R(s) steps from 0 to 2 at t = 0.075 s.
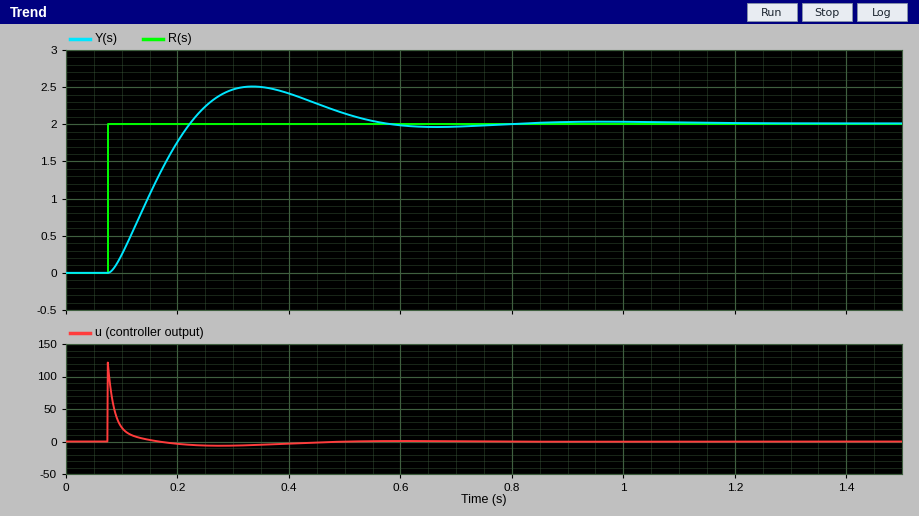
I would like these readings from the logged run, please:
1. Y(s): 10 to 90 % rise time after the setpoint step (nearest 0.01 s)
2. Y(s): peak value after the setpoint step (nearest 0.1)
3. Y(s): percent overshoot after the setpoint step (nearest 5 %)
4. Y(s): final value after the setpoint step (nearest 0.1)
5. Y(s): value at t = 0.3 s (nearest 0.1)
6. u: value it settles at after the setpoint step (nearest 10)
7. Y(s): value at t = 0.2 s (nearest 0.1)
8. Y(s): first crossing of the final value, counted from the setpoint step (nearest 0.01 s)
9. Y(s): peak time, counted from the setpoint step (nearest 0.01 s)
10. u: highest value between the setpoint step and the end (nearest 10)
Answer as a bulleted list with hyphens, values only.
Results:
- 0.11 s
- 2.5
- 25 %
- 2.0
- 2.5
- 0
- 1.8
- 0.15 s
- 0.26 s
- 120
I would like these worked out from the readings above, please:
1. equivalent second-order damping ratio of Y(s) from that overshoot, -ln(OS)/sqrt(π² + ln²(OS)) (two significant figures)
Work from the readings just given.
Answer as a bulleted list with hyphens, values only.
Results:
- 0.40
